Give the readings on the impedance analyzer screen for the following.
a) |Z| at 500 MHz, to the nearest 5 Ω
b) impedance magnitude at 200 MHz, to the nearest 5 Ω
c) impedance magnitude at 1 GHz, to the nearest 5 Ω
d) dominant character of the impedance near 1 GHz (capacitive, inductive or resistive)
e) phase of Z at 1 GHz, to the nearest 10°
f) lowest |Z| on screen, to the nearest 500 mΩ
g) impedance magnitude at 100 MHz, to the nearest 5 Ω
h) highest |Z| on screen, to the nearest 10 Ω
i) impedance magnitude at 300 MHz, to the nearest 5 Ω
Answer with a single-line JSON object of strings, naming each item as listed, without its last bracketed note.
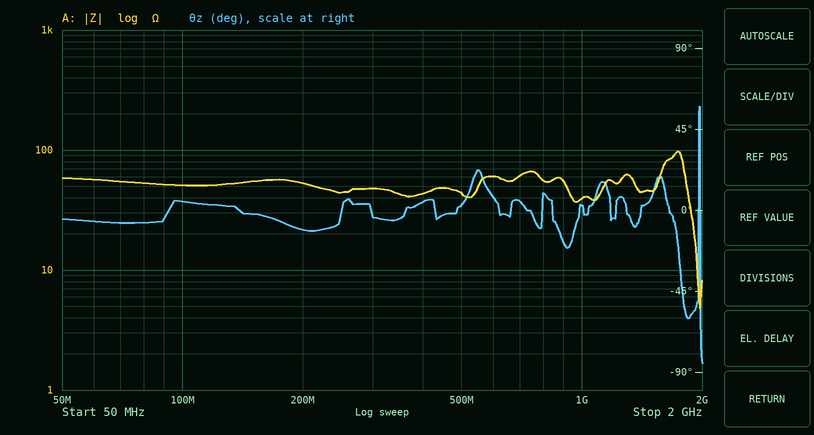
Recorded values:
{"|Z| at 500 MHz, to the nearest 5 Ω": "45 Ω", "impedance magnitude at 200 MHz, to the nearest 5 Ω": "55 Ω", "impedance magnitude at 1 GHz, to the nearest 5 Ω": "40 Ω", "dominant character of the impedance near 1 GHz": "resistive", "phase of Z at 1 GHz, to the nearest 10°": "0°", "lowest |Z| on screen, to the nearest 500 mΩ": "5.0 Ω", "impedance magnitude at 100 MHz, to the nearest 5 Ω": "50 Ω", "highest |Z| on screen, to the nearest 10 Ω": "100 Ω", "impedance magnitude at 300 MHz, to the nearest 5 Ω": "50 Ω"}
